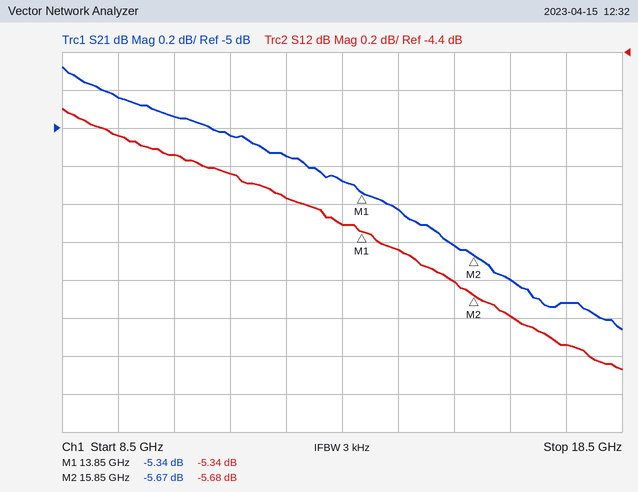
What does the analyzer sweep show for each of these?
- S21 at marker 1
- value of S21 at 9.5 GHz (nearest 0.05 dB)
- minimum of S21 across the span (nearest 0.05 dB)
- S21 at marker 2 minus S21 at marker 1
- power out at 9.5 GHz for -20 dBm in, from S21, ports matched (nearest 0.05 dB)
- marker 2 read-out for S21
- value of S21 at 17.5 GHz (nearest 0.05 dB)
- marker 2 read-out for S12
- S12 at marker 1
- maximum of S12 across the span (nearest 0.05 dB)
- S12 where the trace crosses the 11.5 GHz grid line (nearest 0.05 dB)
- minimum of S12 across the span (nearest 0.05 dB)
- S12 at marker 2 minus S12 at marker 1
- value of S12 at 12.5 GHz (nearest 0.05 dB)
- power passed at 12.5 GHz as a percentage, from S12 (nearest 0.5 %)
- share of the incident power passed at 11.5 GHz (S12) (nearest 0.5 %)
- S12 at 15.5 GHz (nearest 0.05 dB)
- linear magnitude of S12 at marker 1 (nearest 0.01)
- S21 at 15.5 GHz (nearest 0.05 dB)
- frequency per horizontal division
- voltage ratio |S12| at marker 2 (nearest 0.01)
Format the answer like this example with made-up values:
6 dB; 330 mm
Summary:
-5.34 dB; -4.85 dB; -6.05 dB; -0.33 dB; -24.85 dBm; -5.67 dB; -5.90 dB; -5.68 dB; -5.34 dB; -4.70 dB; -5.05 dB; -6.05 dB; -0.34 dB; -5.15 dB; 30.5 %; 31.5 %; -5.60 dB; 0.54; -5.60 dB; 1 GHz; 0.52
